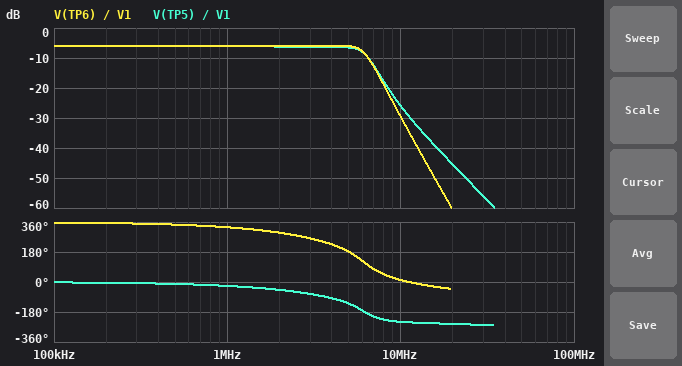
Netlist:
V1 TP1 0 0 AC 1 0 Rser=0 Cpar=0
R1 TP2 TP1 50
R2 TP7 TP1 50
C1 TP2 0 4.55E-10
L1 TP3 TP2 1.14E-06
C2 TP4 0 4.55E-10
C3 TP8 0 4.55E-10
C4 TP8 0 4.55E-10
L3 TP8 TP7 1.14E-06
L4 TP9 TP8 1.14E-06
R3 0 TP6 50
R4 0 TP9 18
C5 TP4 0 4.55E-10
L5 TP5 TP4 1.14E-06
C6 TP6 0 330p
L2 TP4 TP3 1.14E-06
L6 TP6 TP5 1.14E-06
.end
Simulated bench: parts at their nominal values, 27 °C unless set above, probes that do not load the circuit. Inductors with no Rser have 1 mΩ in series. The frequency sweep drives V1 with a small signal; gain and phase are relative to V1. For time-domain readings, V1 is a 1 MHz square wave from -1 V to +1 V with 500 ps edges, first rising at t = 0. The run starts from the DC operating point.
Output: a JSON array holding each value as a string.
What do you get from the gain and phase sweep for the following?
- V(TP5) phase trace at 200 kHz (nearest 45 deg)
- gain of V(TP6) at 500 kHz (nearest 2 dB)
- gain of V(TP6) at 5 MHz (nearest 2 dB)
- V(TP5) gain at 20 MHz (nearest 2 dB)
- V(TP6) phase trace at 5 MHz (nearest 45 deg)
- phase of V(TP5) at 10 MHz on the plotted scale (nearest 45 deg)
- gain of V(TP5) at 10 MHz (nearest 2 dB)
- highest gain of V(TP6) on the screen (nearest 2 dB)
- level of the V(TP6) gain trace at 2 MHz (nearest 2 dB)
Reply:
["0 deg", "-6 dB", "-6 dB", "-46 dB", "180 deg", "-225 deg", "-26 dB", "-6 dB", "-6 dB"]
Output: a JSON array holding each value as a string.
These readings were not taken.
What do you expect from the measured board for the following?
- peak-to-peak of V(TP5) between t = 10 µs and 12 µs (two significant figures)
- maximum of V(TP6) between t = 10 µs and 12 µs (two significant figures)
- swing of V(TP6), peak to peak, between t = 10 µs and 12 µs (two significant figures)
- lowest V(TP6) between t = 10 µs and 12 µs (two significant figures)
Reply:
["1.2 V", "640 mV", "1.3 V", "-640 mV"]
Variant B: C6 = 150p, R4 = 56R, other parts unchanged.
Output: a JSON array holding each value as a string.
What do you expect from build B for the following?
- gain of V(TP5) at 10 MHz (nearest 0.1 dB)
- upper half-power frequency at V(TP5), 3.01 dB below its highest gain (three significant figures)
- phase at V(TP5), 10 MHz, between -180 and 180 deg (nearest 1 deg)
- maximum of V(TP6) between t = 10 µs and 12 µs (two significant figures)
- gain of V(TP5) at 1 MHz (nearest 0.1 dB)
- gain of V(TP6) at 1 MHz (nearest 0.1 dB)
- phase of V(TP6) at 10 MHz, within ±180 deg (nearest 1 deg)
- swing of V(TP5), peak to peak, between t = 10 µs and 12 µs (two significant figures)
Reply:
["-24.8 dB", "6.27 MHz", "118 deg", "630 mV", "-6.0 dB", "-6.0 dB", "41 deg", "1.3 V"]
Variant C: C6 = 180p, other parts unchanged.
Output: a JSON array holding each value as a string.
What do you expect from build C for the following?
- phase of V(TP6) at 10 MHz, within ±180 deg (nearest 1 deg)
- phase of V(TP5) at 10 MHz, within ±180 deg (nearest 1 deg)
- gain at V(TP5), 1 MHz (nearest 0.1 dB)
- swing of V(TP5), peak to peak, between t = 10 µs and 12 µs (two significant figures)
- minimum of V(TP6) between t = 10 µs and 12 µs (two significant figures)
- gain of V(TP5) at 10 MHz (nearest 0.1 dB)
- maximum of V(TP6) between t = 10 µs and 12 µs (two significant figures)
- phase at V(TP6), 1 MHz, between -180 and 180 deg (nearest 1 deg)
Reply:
["35 deg", "118 deg", "-6.0 dB", "1.3 V", "-630 mV", "-25.0 dB", "630 mV", "-30 deg"]
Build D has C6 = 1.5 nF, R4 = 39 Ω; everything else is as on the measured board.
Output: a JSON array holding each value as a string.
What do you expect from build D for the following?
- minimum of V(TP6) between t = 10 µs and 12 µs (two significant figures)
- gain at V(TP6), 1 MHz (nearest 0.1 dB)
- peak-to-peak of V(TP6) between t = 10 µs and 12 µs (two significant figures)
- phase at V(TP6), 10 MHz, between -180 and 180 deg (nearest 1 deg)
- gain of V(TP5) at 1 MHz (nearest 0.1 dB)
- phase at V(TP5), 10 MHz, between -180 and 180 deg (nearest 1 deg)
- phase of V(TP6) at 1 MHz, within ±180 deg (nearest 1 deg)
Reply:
["-570 mV", "-6.1 dB", "1.1 V", "-33 deg", "-6.6 dB", "133 deg", "-42 deg"]
